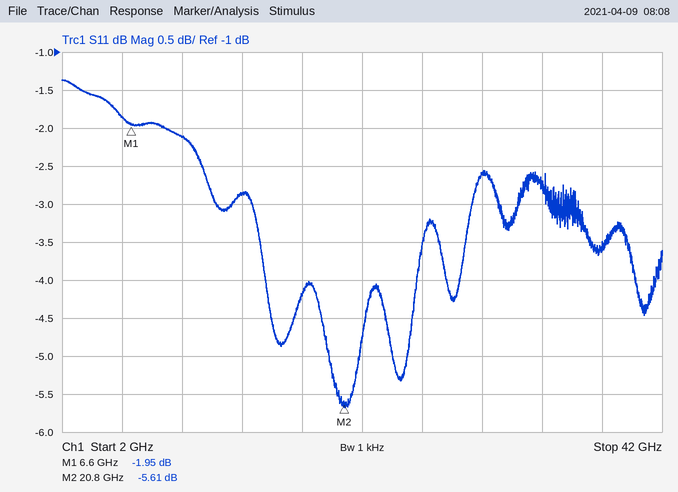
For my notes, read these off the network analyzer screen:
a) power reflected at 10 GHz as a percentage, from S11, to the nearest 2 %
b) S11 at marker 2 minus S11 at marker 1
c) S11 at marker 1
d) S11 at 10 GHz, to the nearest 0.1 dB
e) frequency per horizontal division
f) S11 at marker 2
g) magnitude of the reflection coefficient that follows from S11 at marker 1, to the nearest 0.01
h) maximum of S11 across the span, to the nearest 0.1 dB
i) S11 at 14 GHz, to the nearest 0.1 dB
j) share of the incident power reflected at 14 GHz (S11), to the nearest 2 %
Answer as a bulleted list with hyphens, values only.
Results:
- 62 %
- -3.66 dB
- -1.95 dB
- -2.1 dB
- 4 GHz
- -5.61 dB
- 0.80
- -1.4 dB
- -2.9 dB
- 52 %
